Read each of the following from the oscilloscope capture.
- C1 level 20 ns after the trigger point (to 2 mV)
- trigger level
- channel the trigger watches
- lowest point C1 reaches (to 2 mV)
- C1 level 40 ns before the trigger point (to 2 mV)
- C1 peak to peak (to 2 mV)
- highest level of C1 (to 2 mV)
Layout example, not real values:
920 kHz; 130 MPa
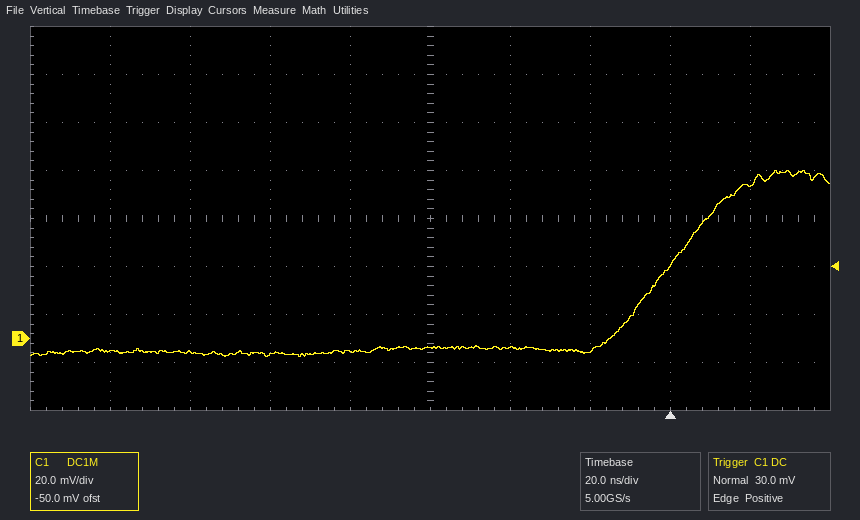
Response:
64 mV; 30.0 mV; C1; -8 mV; -4 mV; 78 mV; 70 mV
